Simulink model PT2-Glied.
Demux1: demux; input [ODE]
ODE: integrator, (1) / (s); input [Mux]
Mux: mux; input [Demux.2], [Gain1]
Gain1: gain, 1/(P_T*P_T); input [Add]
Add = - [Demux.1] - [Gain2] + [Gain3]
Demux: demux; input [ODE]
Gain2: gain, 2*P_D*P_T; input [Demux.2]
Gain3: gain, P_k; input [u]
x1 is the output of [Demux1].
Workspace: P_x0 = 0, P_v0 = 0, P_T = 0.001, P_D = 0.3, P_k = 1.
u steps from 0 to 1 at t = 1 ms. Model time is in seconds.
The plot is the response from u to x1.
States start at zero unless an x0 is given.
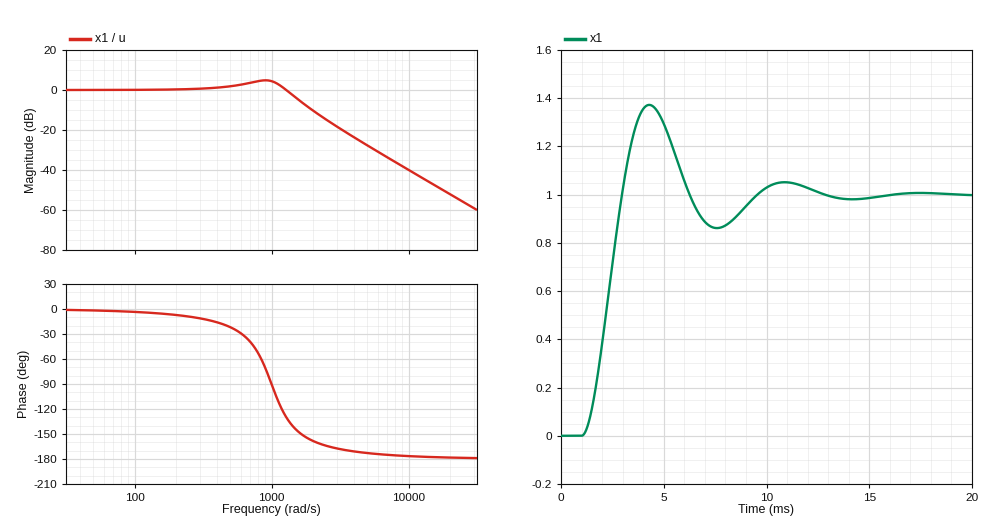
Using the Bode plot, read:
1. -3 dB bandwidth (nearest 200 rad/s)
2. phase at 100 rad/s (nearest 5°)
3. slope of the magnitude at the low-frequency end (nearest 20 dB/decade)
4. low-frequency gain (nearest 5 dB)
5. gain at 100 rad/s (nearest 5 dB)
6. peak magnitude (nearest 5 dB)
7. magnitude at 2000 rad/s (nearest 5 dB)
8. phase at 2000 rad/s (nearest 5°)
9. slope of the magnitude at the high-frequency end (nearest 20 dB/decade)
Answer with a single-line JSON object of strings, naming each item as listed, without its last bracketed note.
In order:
{"-3 dB bandwidth": "1400 rad/s", "phase at 100 rad/s": "-5°", "slope of the magnitude at the low-frequency end": "0 dB/decade", "low-frequency gain": "0 dB", "gain at 100 rad/s": "0 dB", "peak magnitude": "5 dB", "magnitude at 2000 rad/s": "-10 dB", "phase at 2000 rad/s": "-160°", "slope of the magnitude at the high-frequency end": "-40 dB/decade"}
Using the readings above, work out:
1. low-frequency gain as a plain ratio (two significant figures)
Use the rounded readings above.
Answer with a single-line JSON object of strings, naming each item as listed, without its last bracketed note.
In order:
{"low-frequency gain as a plain ratio": "1.0"}
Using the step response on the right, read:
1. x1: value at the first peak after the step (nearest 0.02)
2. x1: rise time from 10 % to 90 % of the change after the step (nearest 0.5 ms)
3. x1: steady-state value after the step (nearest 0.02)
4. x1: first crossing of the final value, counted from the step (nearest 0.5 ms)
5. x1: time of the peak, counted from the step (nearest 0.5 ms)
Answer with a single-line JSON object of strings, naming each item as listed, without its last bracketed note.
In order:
{"x1: value at the first peak after the step": "1.38", "x1: rise time from 10 % to 90 % of the change after the step": "1.5 ms", "x1: steady-state value after the step": "1.00", "x1: first crossing of the final value, counted from the step": "2.0 ms", "x1: time of the peak, counted from the step": "3.5 ms"}
